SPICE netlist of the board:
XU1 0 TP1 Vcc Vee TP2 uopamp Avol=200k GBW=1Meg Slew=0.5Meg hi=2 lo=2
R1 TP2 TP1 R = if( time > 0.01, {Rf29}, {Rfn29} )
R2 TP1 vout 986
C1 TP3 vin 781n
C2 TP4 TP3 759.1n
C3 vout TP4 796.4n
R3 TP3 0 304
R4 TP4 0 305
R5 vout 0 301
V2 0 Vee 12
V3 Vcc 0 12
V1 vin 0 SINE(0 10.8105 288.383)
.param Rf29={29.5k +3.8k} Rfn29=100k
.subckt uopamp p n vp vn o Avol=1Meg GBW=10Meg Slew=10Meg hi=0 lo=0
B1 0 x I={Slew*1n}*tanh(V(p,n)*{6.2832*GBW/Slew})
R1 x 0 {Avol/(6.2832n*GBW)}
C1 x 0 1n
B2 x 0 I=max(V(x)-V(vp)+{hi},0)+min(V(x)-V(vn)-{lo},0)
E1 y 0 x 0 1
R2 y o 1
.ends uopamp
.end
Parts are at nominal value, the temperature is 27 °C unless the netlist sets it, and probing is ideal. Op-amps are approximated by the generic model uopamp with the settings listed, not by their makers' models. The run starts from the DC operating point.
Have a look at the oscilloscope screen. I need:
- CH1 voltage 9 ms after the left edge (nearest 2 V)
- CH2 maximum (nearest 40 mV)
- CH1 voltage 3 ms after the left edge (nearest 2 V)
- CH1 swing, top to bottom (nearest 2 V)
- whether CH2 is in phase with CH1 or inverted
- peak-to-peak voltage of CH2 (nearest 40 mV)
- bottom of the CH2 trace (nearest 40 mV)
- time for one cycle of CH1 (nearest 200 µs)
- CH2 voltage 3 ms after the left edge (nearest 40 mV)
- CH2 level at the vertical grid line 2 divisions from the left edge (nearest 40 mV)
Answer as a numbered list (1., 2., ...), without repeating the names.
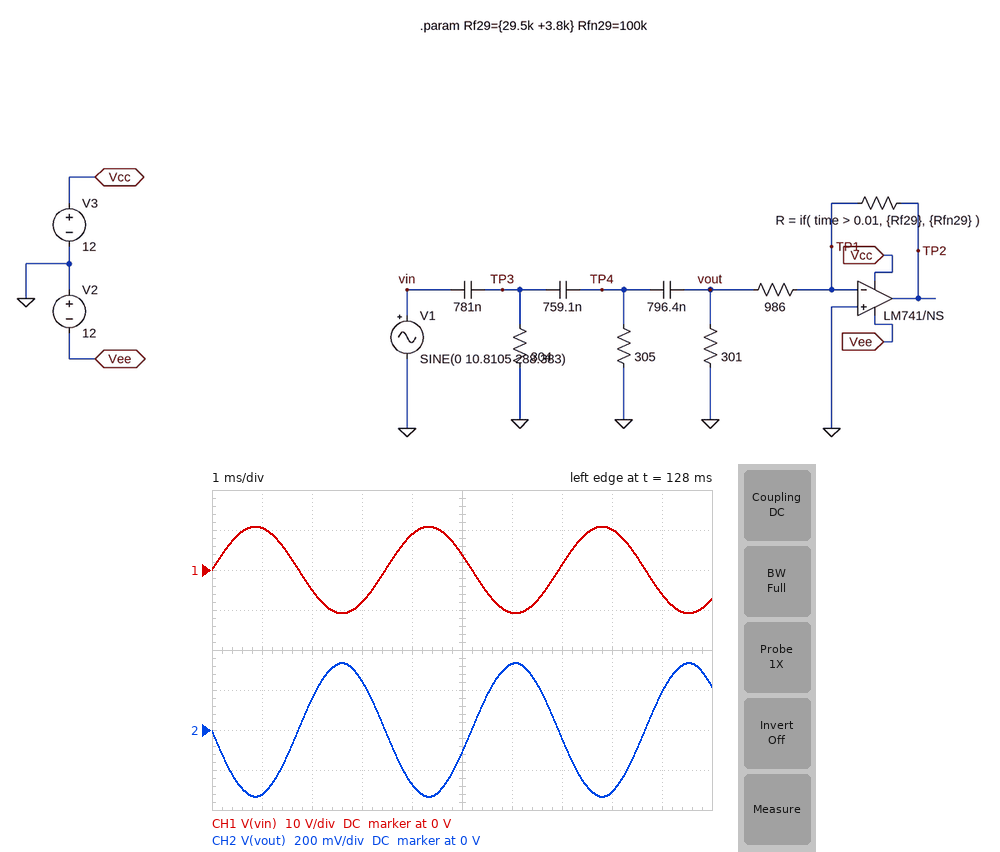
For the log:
1. -6 V
2. 320 mV
3. -8 V
4. 22 V
5. inverted
6. 680 mV
7. -320 mV
8. 3.4 ms
9. 240 mV
10. 160 mV
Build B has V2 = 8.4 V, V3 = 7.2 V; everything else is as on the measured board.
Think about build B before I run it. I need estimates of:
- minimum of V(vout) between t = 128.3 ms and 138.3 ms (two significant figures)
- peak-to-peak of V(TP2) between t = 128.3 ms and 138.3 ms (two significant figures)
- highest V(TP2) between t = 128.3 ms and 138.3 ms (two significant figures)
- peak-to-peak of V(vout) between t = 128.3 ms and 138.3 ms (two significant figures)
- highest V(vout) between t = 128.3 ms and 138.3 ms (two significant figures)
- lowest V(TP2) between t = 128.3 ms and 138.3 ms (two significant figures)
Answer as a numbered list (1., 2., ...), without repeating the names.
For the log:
1. -370 mV
2. 12 V
3. 5.2 V
4. 730 mV
5. 360 mV
6. -6.4 V
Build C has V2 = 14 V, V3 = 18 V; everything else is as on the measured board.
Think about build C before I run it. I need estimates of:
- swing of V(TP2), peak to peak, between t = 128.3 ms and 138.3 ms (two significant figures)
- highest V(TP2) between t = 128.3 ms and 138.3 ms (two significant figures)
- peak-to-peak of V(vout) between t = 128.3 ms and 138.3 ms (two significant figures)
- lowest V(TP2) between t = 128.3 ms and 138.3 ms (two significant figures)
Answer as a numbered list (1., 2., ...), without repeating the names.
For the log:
1. 22 V
2. 11 V
3. 660 mV
4. -11 V
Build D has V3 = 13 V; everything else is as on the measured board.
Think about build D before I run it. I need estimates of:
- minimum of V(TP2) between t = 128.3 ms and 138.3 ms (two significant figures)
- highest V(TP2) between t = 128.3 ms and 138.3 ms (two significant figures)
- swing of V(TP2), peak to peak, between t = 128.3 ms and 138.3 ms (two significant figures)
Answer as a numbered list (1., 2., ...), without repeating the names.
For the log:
1. -10 V
2. 11 V
3. 21 V
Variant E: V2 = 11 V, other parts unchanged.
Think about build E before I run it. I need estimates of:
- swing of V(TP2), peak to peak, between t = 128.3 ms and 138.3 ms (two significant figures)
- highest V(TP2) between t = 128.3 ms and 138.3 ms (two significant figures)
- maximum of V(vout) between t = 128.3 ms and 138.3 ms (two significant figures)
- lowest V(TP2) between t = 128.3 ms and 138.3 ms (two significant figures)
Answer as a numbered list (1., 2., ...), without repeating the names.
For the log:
1. 19 V
2. 10 V
3. 340 mV
4. -9.0 V
